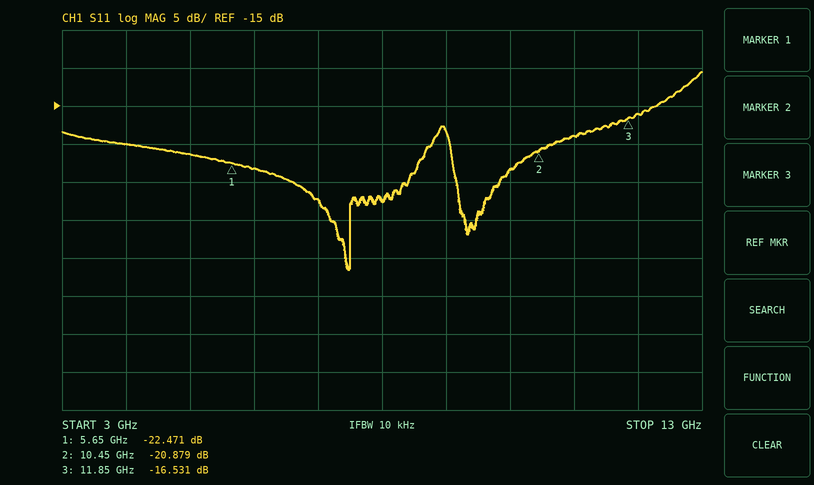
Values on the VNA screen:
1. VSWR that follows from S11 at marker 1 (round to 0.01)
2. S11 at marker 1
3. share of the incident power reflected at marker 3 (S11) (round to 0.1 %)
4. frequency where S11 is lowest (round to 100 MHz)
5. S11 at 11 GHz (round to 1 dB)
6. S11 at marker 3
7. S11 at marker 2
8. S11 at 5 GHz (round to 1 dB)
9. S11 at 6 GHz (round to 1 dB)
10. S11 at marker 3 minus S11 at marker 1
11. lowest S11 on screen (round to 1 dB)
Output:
1.16
-22.471 dB
2.2 %
7.5 GHz
-19 dB
-16.531 dB
-20.879 dB
-21 dB
-23 dB
5.940 dB
-37 dB
